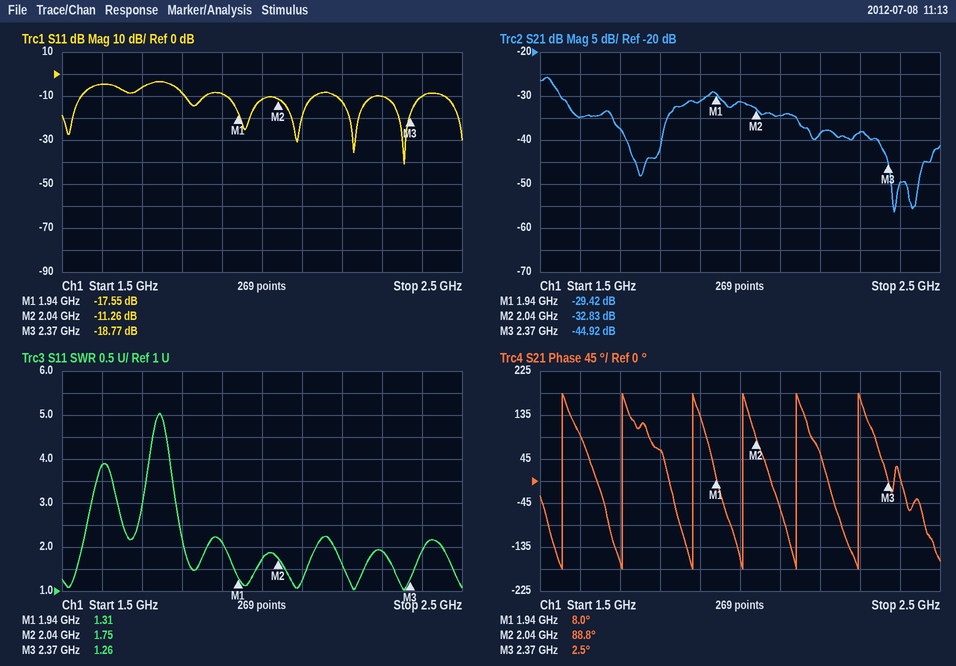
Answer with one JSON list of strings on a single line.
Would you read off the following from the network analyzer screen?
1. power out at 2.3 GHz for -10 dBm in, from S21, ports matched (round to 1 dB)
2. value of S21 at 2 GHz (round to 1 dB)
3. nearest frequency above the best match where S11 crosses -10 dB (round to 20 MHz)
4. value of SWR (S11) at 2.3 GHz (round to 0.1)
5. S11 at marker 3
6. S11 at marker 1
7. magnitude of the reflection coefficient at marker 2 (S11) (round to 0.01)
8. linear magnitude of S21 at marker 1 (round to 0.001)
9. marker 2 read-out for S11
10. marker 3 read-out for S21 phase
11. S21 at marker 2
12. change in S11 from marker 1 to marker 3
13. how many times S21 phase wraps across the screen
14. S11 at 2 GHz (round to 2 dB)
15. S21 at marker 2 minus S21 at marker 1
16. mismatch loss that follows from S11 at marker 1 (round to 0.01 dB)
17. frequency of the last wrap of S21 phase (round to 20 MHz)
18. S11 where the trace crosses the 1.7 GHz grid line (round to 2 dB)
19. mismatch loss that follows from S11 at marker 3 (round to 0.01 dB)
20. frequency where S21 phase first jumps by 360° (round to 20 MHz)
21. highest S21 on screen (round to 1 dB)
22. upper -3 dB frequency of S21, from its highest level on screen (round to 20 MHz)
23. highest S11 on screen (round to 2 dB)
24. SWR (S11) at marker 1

["-48 dBm", "-31 dB", "2.40 GHz", "1.9", "-18.77 dB", "-17.55 dB", "0.27", "0.034", "-11.26 dB", "2.5°", "-32.83 dB", "-1.22 dB", "6", "-12 dB", "-3.41 dB", "0.08 dB", "2.30 GHz", "-6 dB", "0.06 dB", "1.56 GHz", "-26 dB", "1.54 GHz", "-4 dB", "1.31"]
